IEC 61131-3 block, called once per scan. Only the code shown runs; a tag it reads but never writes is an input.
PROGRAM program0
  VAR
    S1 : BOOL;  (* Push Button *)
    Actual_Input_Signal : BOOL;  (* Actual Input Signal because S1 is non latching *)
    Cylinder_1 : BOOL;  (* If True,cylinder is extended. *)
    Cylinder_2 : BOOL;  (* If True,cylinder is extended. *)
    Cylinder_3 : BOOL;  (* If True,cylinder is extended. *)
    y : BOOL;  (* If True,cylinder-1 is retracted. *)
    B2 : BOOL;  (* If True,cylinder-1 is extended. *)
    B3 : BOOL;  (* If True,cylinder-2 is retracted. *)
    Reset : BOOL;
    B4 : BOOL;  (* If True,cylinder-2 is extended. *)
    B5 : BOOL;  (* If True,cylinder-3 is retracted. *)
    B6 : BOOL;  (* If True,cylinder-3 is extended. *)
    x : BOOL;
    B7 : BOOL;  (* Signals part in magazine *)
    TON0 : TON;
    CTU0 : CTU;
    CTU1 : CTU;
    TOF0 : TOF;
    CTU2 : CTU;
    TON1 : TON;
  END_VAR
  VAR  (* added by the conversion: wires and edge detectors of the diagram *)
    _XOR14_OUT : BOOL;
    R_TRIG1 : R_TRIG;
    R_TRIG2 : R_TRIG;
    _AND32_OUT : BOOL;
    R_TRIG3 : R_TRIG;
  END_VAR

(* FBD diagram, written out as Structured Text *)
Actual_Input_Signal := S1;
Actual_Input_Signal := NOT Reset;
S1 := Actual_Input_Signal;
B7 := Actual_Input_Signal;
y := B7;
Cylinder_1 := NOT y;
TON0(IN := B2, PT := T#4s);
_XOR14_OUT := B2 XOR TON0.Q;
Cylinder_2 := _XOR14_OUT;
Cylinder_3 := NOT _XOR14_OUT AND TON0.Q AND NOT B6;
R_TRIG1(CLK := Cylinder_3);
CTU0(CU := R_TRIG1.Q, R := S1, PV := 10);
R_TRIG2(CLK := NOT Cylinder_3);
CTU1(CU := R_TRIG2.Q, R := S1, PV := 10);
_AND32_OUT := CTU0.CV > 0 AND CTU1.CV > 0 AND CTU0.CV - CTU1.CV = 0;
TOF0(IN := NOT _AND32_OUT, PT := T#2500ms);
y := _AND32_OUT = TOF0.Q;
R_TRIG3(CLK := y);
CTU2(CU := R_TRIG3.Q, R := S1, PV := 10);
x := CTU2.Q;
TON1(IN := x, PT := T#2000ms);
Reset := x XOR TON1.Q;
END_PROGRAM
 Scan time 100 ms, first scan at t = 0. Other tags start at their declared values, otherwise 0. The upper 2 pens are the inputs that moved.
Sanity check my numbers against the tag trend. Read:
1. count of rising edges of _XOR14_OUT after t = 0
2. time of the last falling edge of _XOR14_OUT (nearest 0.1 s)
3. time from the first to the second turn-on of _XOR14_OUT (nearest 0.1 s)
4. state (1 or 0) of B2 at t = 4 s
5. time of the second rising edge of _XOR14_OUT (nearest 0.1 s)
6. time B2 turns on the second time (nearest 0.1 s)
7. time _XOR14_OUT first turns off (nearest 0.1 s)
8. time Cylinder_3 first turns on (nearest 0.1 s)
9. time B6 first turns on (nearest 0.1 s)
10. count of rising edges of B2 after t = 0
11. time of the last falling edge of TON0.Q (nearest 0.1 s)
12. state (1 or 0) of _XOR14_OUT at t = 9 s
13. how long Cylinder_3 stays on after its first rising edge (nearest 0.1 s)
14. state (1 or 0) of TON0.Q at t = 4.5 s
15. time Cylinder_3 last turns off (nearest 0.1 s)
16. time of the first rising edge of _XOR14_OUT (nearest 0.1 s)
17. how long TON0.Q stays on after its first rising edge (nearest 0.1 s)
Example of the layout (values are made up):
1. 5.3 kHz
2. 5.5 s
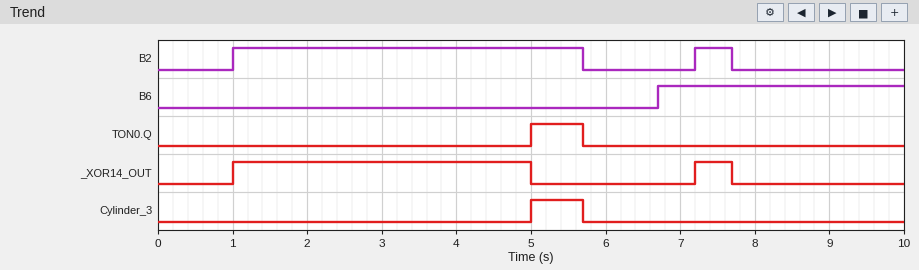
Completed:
1. 2
2. 7.7 s
3. 6.2 s
4. 1
5. 7.2 s
6. 7.2 s
7. 5.0 s
8. 5.0 s
9. 6.7 s
10. 2
11. 5.7 s
12. 0
13. 0.7 s
14. 0
15. 5.7 s
16. 1.0 s
17. 0.7 s
